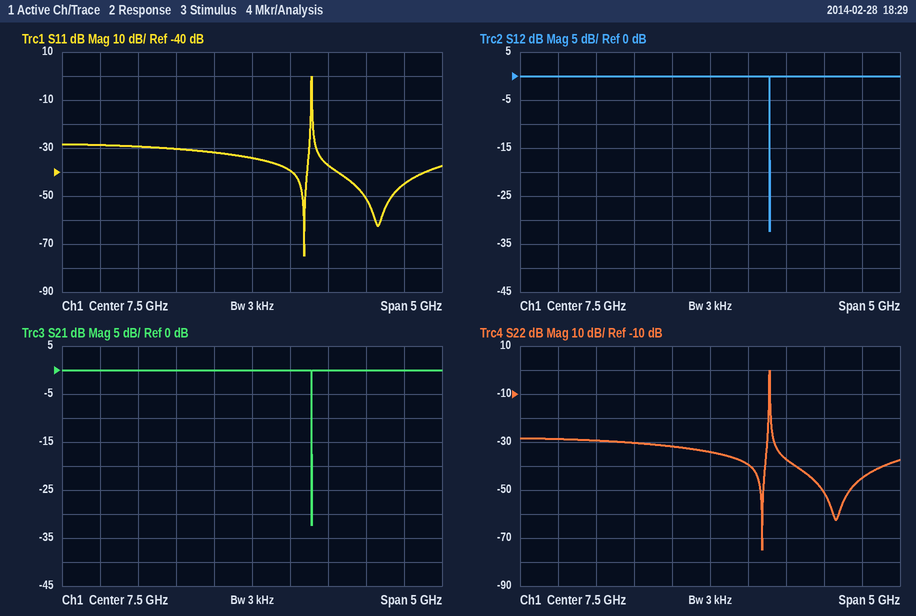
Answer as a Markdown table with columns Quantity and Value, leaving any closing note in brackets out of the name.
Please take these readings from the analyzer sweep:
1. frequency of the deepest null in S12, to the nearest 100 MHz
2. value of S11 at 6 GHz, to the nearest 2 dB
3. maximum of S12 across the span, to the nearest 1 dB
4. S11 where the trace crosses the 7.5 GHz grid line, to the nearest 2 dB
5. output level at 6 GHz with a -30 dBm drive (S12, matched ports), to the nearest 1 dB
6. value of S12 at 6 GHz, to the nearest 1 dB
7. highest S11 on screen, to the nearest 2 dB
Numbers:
| Quantity | Value |
|---|---|
| frequency of the deepest null in S12, to the nearest 100 MHz | 8.3 GHz |
| value of S11 at 6 GHz, to the nearest 2 dB | -30 dB |
| maximum of S12 across the span, to the nearest 1 dB | 0 dB |
| S11 where the trace crosses the 7.5 GHz grid line, to the nearest 2 dB | -34 dB |
| output level at 6 GHz with a -30 dBm drive (S12, matched ports), to the nearest 1 dB | -30 dBm |
| value of S12 at 6 GHz, to the nearest 1 dB | 0 dB |
| highest S11 on screen, to the nearest 2 dB | 0 dB |
